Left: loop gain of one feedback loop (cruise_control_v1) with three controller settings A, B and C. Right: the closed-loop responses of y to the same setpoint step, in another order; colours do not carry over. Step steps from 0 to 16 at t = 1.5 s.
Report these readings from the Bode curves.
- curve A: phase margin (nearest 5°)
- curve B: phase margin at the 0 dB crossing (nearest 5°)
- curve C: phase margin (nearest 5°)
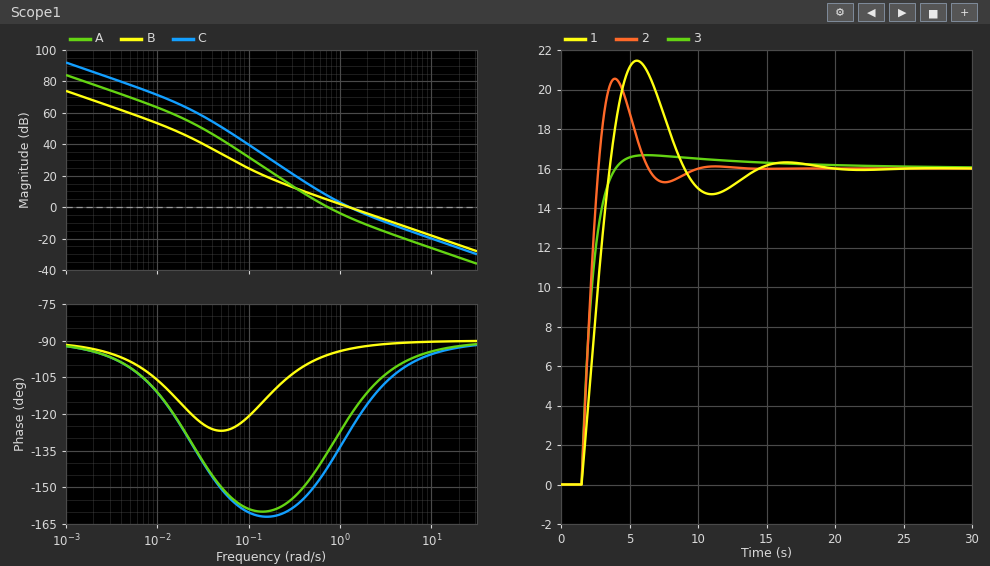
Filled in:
45°
85°
55°
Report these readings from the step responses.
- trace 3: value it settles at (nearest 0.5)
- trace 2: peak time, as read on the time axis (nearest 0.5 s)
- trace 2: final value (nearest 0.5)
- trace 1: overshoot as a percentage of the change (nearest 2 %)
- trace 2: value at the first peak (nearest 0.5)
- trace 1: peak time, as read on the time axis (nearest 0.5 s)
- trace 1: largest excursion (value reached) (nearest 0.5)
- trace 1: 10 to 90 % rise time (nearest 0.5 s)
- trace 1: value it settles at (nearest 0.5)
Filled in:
16.0
4.0 s
16.0
34 %
20.5
5.5 s
21.5
1.5 s
16.0
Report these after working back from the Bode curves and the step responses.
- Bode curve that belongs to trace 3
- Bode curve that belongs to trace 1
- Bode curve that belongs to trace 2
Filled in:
B
A
C
